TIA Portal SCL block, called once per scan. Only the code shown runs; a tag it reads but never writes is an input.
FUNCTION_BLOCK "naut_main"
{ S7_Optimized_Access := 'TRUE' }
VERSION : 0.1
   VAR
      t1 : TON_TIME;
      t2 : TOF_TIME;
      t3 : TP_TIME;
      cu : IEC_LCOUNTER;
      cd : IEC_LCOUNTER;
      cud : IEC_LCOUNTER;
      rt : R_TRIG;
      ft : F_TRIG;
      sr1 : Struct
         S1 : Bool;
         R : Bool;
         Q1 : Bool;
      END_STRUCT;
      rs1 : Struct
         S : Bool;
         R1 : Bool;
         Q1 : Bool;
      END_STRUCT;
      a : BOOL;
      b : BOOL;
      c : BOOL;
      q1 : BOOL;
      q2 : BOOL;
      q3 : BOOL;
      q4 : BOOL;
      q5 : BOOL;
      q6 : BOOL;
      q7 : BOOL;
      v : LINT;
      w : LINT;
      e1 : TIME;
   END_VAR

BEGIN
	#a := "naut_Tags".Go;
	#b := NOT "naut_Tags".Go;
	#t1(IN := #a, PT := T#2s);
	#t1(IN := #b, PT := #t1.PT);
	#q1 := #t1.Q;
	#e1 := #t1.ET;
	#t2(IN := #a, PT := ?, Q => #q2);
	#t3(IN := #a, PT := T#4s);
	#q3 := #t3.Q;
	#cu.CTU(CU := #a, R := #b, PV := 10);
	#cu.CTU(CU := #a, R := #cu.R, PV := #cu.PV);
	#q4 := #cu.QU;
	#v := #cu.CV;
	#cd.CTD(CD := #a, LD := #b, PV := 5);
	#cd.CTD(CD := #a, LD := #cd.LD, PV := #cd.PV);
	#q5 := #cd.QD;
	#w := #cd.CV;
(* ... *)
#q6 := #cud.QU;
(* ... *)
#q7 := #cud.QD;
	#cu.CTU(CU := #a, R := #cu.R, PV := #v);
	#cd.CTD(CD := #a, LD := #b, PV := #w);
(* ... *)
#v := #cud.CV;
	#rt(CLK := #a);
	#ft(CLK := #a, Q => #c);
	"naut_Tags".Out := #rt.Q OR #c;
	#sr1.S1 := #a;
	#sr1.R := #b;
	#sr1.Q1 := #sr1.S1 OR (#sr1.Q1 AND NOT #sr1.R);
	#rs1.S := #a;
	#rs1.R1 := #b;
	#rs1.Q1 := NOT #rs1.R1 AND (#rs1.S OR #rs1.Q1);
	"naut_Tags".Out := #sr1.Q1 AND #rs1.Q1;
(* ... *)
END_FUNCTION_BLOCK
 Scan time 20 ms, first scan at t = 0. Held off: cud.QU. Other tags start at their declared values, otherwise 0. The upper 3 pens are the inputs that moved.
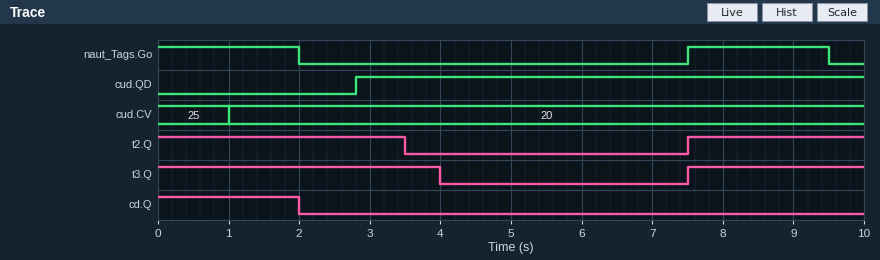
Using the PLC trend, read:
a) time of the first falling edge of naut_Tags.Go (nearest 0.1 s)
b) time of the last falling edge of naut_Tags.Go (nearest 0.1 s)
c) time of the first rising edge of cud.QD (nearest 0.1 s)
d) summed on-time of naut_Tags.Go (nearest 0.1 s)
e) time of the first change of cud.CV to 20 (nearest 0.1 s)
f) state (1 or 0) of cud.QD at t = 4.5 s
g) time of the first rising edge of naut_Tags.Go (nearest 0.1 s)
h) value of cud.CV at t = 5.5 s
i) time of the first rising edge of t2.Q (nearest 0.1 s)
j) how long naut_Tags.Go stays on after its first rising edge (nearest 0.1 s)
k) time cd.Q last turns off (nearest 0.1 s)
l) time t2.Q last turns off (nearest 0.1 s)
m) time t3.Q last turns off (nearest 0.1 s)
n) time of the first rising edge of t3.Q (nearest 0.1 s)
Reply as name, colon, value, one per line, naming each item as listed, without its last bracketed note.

time of the first falling edge of naut_Tags.Go: 2.0 s
time of the last falling edge of naut_Tags.Go: 9.5 s
time of the first rising edge of cud.QD: 2.8 s
summed on-time of naut_Tags.Go: 4.0 s
time of the first change of cud.CV to 20: 1.0 s
state (1 or 0) of cud.QD at t = 4.5 s: 1
time of the first rising edge of naut_Tags.Go: 7.5 s
value of cud.CV at t = 5.5 s: 20
time of the first rising edge of t2.Q: 7.5 s
how long naut_Tags.Go stays on after its first rising edge: 2.0 s
time cd.Q last turns off: 2.0 s
time t2.Q last turns off: 3.5 s
time t3.Q last turns off: 4.0 s
time of the first rising edge of t3.Q: 7.5 s
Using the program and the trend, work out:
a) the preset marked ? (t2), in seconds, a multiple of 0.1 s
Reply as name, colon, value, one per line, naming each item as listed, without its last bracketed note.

the preset marked ? (t2), in seconds, a multiple of 0.1 s: 1.5 s
